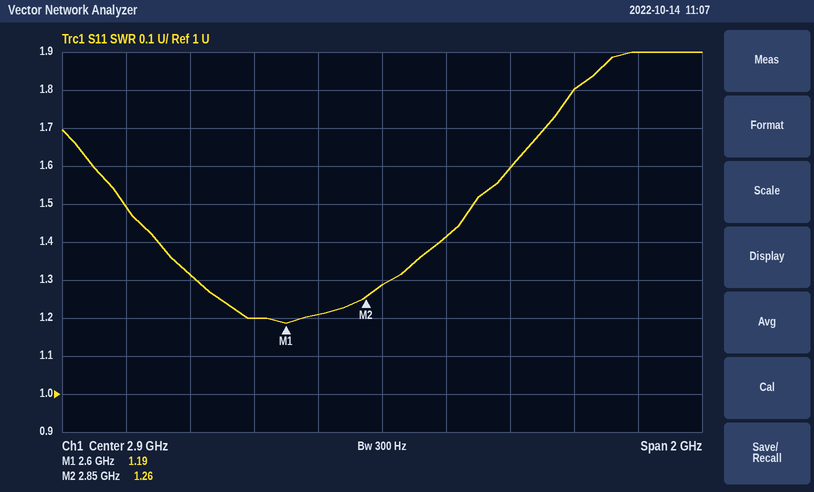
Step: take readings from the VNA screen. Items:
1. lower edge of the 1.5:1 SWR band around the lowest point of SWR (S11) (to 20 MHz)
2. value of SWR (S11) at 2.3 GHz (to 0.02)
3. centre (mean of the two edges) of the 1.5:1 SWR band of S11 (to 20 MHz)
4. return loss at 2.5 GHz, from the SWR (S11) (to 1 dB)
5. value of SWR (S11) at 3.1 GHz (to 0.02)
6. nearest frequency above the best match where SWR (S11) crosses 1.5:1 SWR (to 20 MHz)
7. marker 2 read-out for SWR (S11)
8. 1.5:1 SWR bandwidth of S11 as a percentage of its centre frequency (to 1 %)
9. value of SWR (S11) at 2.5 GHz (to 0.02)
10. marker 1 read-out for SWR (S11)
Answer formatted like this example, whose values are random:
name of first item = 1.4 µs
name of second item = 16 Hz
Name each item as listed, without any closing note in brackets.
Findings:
lower edge of the 1.5:1 SWR band around the lowest point of SWR (S11) = 2.10 GHz
value of SWR (S11) at 2.3 GHz = 1.32
centre (mean of the two edges) of the 1.5:1 SWR band of S11 = 2.64 GHz
return loss at 2.5 GHz, from the SWR (S11) = 21 dB
value of SWR (S11) at 3.1 GHz = 1.42
nearest frequency above the best match where SWR (S11) crosses 1.5:1 SWR = 3.18 GHz
marker 2 read-out for SWR = 1.26
1.5:1 SWR bandwidth of S11 as a percentage of its centre frequency = 41 %
value of SWR (S11) at 2.5 GHz = 1.20
marker 1 read-out for SWR = 1.19
